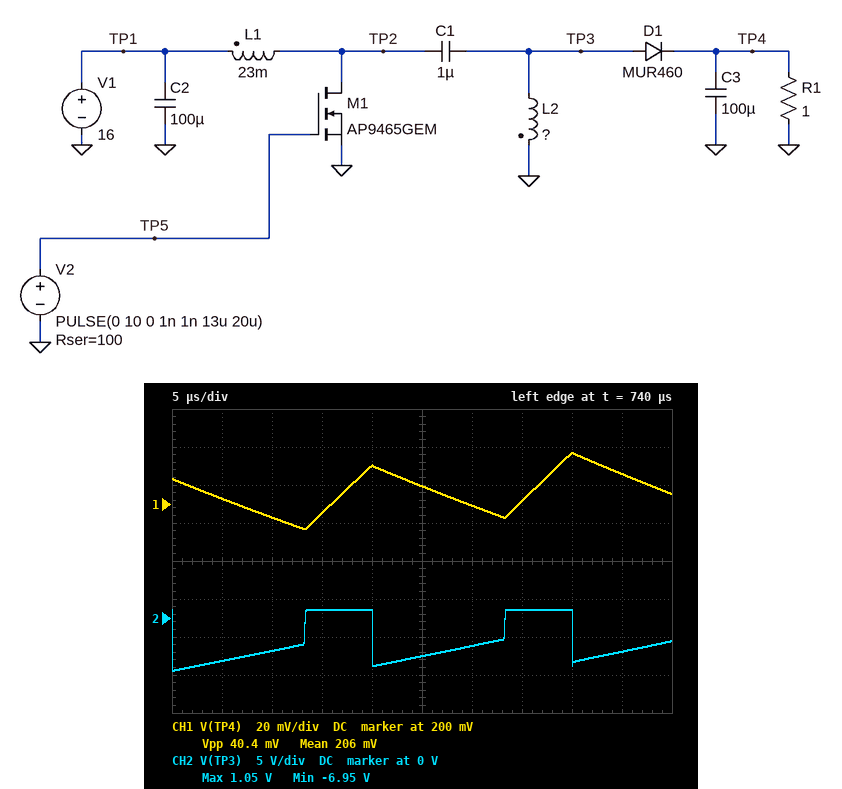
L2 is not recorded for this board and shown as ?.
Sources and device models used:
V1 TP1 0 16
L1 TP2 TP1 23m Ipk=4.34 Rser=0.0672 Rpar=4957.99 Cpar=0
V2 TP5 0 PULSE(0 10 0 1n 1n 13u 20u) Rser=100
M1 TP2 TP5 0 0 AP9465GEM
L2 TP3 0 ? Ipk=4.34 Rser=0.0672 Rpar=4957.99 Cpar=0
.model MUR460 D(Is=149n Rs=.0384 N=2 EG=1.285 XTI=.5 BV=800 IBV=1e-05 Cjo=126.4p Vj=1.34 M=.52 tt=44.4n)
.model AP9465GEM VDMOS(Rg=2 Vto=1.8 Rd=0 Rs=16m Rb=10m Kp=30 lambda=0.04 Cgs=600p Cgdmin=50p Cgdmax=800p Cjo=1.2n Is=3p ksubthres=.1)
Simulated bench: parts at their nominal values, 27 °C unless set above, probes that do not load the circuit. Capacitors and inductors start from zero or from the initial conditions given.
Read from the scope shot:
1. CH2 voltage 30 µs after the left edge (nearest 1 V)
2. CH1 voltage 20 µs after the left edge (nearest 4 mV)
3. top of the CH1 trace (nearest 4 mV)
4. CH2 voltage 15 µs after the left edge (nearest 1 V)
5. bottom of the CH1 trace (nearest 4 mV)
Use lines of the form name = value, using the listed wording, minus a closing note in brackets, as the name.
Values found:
CH2 voltage 30 µs after the left edge = -4 V
CH1 voltage 20 µs after the left edge = 220 mV
top of the CH1 trace = 228 mV
CH2 voltage 15 µs after the left edge = 1 V
bottom of the CH1 trace = 188 mV
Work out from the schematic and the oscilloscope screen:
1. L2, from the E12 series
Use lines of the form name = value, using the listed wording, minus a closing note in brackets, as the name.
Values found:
L2, from the E12 series = 12 mH
